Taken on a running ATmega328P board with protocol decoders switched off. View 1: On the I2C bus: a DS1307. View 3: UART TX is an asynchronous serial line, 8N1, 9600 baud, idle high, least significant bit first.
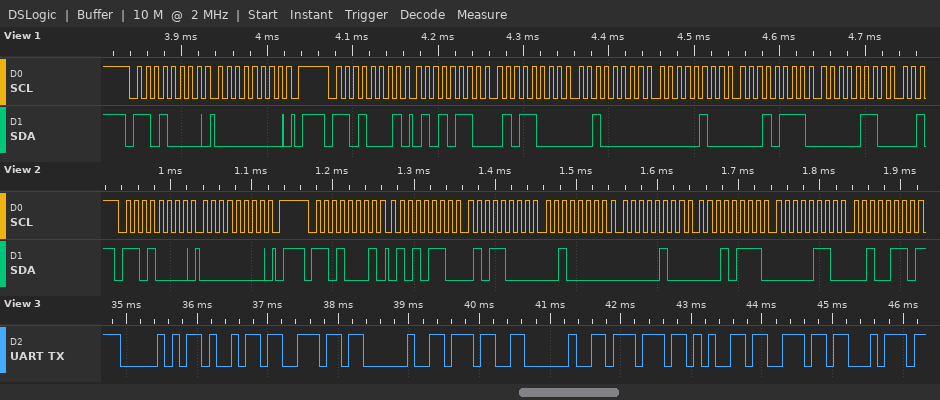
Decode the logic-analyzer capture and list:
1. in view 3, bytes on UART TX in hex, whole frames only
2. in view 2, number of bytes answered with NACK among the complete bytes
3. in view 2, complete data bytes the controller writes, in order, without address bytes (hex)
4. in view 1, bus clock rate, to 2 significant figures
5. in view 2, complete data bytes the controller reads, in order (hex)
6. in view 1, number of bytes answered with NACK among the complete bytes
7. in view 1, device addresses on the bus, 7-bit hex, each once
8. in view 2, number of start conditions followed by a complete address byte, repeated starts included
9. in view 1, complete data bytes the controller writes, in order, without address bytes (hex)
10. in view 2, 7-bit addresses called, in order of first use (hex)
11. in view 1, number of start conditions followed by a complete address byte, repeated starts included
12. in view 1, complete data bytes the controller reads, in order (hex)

0x50 0x69 0x6E 0x20 0x37 0x20 0x77 0x65 0x6E 0x74
1
00
100 kHz
56 58 20 04 17 06 26
0
0x68
2
00
0x68
2
56 58 20 04 17 06
